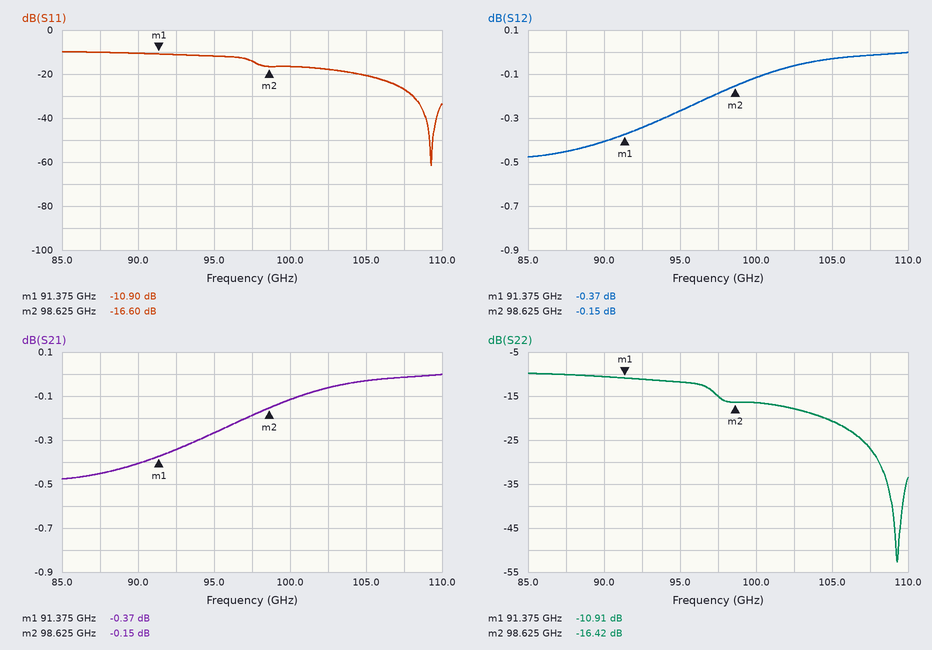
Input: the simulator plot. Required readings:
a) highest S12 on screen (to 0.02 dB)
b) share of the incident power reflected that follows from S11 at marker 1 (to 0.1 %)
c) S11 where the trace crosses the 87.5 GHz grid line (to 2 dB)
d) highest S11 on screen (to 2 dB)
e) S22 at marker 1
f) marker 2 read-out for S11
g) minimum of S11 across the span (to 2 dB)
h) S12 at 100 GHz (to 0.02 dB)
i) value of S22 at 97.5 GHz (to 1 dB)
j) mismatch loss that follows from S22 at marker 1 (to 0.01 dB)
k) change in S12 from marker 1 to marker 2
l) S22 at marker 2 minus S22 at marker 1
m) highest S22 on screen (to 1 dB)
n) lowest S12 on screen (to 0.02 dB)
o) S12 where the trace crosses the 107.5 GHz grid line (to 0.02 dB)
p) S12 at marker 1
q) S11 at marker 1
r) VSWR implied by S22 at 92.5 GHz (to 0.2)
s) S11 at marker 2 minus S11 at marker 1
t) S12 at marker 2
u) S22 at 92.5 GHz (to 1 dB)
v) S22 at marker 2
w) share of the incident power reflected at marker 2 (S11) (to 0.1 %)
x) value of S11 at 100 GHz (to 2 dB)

0.00 dB
8.1 %
-10 dB
-10 dB
-10.91 dB
-16.60 dB
-62 dB
-0.12 dB
-15 dB
0.37 dB
0.22 dB
-5.51 dB
-10 dB
-0.48 dB
-0.02 dB
-0.37 dB
-10.90 dB
1.8
-5.70 dB
-0.15 dB
-11 dB
-16.42 dB
2.2 %
-16 dB
